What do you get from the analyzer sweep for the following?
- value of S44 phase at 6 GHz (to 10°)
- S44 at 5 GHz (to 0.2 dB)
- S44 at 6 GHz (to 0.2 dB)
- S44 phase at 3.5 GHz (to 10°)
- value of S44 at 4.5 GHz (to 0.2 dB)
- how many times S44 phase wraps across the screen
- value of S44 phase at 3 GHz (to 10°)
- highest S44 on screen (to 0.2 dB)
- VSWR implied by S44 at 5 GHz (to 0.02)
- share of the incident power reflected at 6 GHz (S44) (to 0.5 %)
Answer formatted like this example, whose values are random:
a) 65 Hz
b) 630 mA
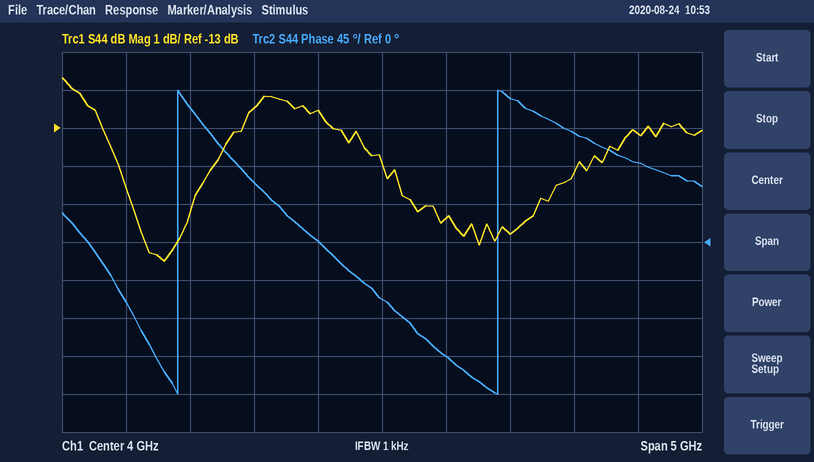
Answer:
a) 90°
b) -15.8 dB
c) -13.2 dB
d) 0°
e) -15.4 dB
f) 2
g) 70°
h) -11.6 dB
i) 1.38
j) 5.0 %
